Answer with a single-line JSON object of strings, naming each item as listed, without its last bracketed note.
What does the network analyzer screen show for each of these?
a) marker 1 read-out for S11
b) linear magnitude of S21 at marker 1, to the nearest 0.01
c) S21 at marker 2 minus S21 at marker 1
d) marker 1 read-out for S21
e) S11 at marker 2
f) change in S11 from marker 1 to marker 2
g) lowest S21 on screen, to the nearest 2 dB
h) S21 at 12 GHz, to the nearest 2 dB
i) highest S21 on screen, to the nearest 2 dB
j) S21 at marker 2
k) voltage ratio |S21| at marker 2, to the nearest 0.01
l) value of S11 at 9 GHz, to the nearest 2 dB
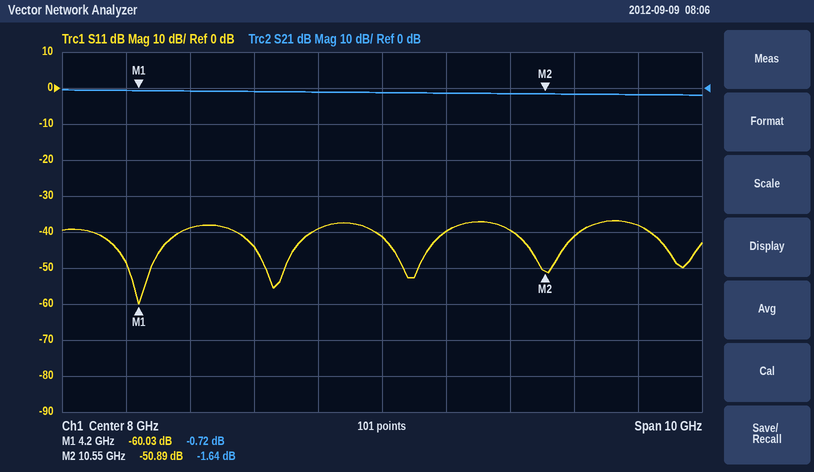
{"marker 1 read-out for S11": "-60.03 dB", "linear magnitude of S21 at marker 1, to the nearest 0.01": "0.92", "S21 at marker 2 minus S21 at marker 1": "-0.92 dB", "marker 1 read-out for S21": "-0.72 dB", "S11 at marker 2": "-50.89 dB", "change in S11 from marker 1 to marker 2": "9.14 dB", "lowest S21 on screen, to the nearest 2 dB": "-2 dB", "S21 at 12 GHz, to the nearest 2 dB": "-2 dB", "highest S21 on screen, to the nearest 2 dB": "0 dB", "S21 at marker 2": "-1.64 dB", "voltage ratio |S21| at marker 2, to the nearest 0.01": "0.83", "value of S11 at 9 GHz, to the nearest 2 dB": "-40 dB"}
